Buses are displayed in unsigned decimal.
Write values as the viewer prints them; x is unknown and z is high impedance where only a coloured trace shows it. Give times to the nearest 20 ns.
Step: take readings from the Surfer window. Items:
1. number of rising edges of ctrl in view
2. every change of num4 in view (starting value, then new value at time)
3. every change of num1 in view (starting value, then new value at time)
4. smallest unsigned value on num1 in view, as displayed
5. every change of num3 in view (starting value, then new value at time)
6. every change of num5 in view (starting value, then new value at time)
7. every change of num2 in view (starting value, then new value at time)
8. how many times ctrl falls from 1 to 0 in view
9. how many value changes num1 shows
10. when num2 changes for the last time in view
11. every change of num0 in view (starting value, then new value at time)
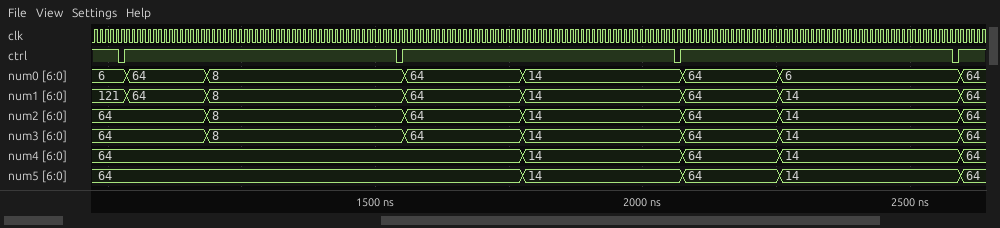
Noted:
4
64, 14 at 1780 ns, 64 at 2080 ns, 14 at 2260 ns, 64 at 2600 ns
121, 64 at 1040 ns, 8 at 1180 ns, 64 at 1560 ns, 14 at 1780 ns, 64 at 2080 ns, 14 at 2260 ns, 64 at 2600 ns
8
64, 8 at 1180 ns, 64 at 1560 ns, 14 at 1780 ns, 64 at 2080 ns, 14 at 2260 ns, 64 at 2600 ns
64, 14 at 1780 ns, 64 at 2080 ns, 14 at 2260 ns, 64 at 2600 ns
64, 8 at 1180 ns, 64 at 1560 ns, 14 at 1780 ns, 64 at 2080 ns, 14 at 2260 ns, 64 at 2600 ns
4
7
2600 ns
6, 64 at 1040 ns, 8 at 1180 ns, 64 at 1560 ns, 14 at 1780 ns, 64 at 2080 ns, 6 at 2260 ns, 64 at 2600 ns
